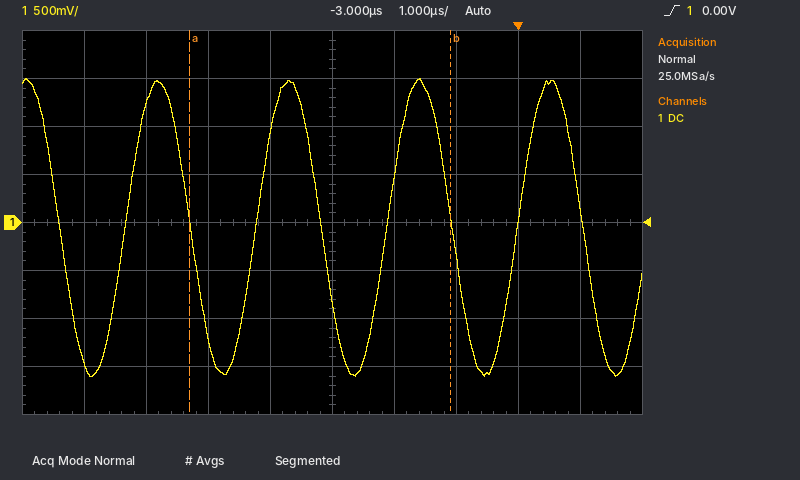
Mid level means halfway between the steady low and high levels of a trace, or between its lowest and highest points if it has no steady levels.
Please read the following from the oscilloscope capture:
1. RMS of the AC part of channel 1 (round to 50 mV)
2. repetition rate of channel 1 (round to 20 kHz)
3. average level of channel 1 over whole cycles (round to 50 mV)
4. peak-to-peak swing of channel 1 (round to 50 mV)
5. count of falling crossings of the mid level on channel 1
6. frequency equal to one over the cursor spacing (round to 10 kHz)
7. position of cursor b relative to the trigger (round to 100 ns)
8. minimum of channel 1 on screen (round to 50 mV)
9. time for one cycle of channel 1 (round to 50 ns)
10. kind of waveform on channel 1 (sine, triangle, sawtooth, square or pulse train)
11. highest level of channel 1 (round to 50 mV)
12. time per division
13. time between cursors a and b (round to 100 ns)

1.10 V
480 kHz
-50 mV
3.10 V
5
240 kHz
-1.1 µs
-1.60 V
2.10 µs
sine
1.50 V
1 µs
4.2 µs
